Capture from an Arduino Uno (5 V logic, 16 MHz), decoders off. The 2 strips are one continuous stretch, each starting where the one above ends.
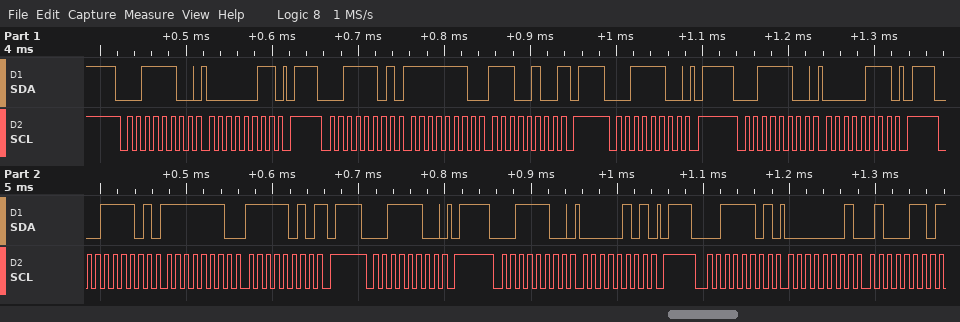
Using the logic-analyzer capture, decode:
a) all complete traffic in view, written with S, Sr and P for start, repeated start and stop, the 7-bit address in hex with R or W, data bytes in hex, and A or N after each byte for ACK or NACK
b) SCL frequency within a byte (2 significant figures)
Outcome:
S 1EW A 03 A P S 1ER A FE A E4 N P S 1EW A P S 1EW A 07 A P S 1ER A FE A FA N P S 1EW A P S 1EW A 05 A P S 1ER A 01 A 46 N
100 kHz
